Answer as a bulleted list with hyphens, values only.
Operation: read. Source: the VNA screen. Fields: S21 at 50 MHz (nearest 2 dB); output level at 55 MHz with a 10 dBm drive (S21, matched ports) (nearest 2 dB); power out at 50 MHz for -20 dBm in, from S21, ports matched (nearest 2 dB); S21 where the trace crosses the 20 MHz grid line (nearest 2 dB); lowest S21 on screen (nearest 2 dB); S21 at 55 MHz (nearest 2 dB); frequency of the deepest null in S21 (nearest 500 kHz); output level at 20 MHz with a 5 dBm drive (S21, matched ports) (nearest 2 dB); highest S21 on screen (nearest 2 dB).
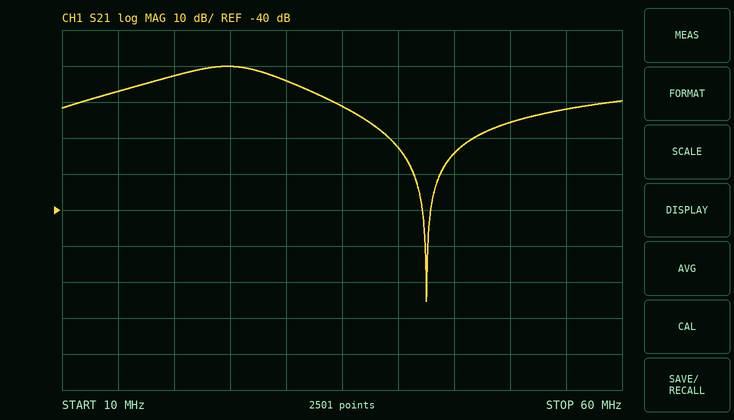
- -16 dB
- -2 dBm
- -36 dBm
- -2 dB
- -66 dB
- -12 dB
- 42.5 MHz
- 2 dBm
- 0 dB
